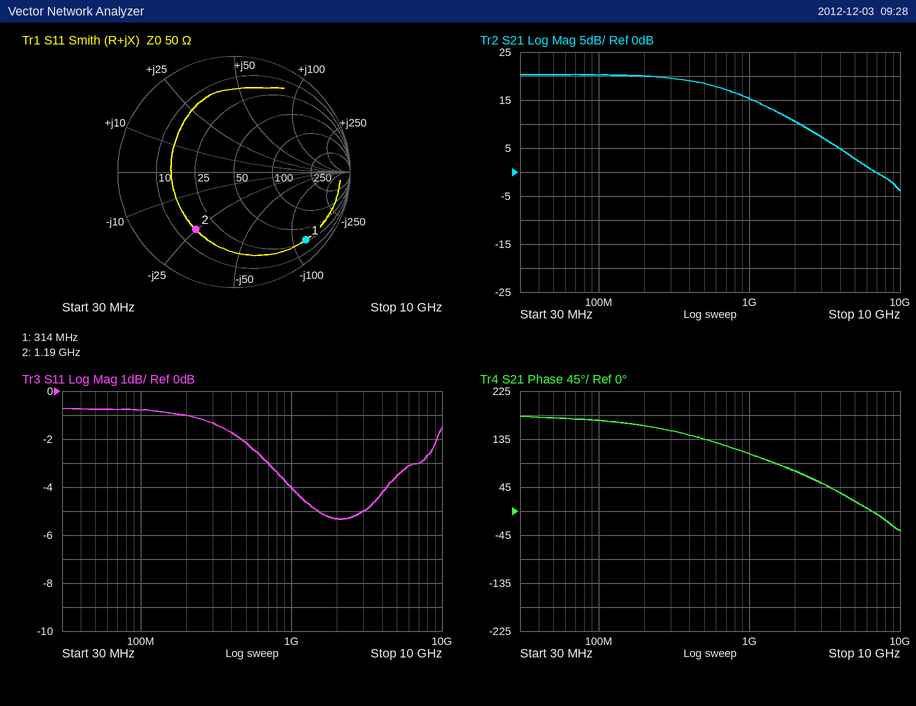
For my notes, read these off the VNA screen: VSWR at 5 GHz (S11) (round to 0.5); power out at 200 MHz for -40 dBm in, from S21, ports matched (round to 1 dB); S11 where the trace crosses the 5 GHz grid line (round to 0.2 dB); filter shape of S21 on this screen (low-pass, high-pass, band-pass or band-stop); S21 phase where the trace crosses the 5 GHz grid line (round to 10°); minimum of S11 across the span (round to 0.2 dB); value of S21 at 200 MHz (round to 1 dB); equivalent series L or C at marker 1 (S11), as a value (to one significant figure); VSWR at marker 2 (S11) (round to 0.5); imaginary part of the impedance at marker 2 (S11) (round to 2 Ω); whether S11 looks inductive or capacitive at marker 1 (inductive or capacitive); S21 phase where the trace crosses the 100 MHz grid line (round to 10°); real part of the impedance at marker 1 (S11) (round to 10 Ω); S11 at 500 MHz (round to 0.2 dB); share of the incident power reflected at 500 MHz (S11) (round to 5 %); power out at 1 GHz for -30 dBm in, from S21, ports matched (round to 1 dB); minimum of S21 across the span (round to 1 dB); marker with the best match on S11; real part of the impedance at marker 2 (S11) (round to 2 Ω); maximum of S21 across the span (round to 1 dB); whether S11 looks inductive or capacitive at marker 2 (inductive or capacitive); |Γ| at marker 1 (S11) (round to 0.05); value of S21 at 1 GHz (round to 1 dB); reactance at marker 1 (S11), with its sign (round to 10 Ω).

5.0
-20 dBm
-3.6 dB
low-pass
20°
-5.4 dB
20 dB
4 pF
4.0
-24 Ω
capacitive
170°
30 Ω
-2.2 dB
60 %
-15 dBm
-4 dB
marker 2
16 Ω
20 dB
capacitive
0.85
15 dB
-120 Ω
